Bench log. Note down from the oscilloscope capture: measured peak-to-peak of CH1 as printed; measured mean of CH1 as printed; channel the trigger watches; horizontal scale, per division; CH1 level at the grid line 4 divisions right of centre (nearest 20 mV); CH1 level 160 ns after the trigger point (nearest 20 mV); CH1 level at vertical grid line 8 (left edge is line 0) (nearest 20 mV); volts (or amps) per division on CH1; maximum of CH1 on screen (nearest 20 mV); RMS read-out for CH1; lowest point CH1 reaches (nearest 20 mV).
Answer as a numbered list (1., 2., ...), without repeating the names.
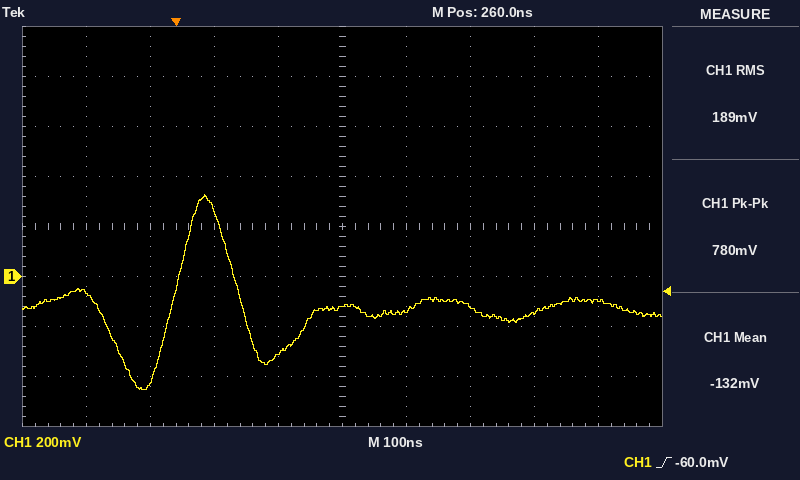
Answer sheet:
1. 780 mV
2. -132 mV
3. CH1
4. 100 ns
5. -100 mV
6. -300 mV
7. -140 mV
8. 200 mV
9. 320 mV
10. 189 mV
11. -460 mV
